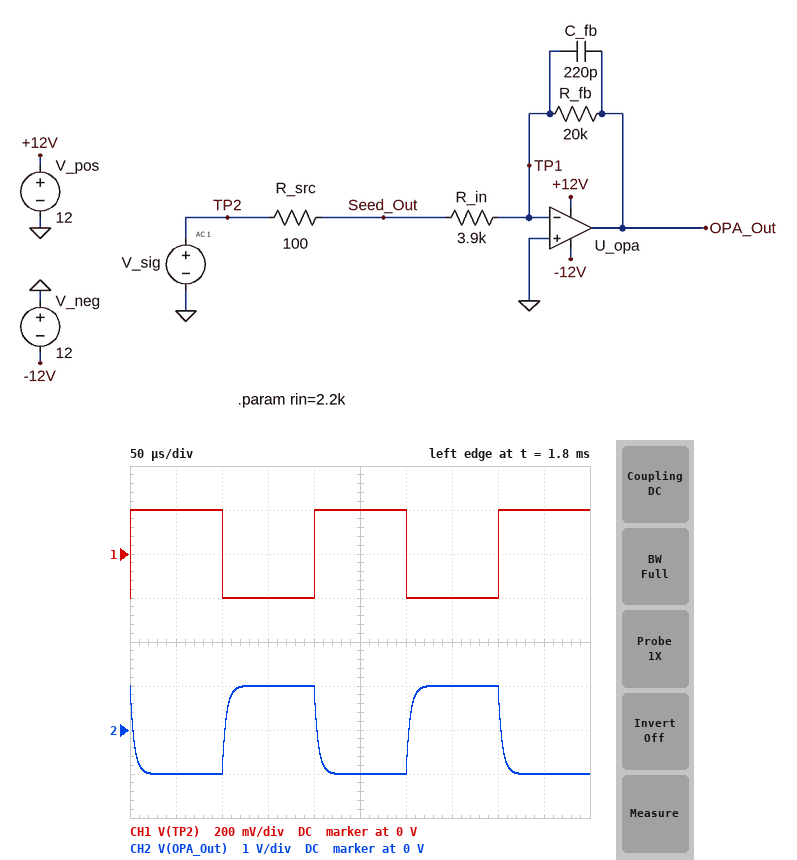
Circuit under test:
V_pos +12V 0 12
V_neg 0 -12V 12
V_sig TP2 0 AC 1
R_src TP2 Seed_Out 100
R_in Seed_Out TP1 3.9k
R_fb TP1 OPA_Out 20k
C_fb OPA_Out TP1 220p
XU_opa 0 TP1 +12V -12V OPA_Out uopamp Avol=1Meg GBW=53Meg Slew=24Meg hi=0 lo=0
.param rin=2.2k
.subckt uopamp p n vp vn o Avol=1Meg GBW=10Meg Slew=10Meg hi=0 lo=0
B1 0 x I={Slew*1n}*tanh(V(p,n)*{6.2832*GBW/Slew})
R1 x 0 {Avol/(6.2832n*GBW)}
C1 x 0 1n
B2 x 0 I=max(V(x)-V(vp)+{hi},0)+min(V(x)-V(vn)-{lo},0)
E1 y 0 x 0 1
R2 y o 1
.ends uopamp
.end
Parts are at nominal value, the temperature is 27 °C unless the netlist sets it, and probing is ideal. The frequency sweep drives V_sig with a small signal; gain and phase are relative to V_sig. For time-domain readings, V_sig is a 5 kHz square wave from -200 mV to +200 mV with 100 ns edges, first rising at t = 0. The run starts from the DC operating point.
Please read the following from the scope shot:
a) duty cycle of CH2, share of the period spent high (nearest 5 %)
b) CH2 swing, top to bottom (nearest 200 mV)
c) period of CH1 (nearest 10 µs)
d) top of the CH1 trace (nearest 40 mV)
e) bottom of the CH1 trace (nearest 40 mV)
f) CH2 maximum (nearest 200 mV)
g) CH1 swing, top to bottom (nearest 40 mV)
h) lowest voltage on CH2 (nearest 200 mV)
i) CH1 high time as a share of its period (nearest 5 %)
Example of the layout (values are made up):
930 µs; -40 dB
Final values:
50 %; 2.0 V; 200 µs; 200 mV; -200 mV; 1.0 V; 400 mV; -1.0 V; 50 %
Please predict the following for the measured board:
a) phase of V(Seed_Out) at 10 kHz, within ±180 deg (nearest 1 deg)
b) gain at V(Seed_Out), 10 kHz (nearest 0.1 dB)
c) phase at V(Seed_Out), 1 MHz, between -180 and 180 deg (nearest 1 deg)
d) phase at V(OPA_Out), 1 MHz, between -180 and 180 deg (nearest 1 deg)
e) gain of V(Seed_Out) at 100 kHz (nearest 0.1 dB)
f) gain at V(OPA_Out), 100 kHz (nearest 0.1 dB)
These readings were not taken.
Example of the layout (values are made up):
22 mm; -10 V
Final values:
0 deg; -0.2 dB; 0 deg; 91 deg; -0.2 dB; 4.6 dB
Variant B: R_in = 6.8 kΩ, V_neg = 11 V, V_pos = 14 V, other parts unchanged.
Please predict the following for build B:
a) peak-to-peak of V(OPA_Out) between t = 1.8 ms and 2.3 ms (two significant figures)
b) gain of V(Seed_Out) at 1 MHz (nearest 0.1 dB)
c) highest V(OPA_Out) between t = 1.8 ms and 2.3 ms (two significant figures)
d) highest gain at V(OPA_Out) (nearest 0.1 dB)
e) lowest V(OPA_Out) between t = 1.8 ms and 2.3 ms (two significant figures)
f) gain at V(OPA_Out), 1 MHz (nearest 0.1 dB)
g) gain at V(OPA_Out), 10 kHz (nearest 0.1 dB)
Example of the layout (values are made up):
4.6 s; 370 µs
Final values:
1.2 V; -0.1 dB; 580 mV; 9.2 dB; -580 mV; -19.6 dB; 8.9 dB
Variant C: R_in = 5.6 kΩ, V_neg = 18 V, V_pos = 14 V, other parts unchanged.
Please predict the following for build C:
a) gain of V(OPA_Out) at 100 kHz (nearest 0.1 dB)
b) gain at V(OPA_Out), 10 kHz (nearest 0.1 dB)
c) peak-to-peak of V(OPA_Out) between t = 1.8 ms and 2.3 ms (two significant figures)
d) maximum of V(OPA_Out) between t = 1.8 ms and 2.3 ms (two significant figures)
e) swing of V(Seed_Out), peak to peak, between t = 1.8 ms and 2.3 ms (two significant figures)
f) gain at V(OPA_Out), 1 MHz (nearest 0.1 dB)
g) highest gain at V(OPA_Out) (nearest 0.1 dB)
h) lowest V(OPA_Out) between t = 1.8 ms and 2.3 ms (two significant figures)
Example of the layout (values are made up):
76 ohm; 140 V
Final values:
1.5 dB; 10.6 dB; 1.4 V; 700 mV; 390 mV; -18.0 dB; 10.9 dB; -700 mV
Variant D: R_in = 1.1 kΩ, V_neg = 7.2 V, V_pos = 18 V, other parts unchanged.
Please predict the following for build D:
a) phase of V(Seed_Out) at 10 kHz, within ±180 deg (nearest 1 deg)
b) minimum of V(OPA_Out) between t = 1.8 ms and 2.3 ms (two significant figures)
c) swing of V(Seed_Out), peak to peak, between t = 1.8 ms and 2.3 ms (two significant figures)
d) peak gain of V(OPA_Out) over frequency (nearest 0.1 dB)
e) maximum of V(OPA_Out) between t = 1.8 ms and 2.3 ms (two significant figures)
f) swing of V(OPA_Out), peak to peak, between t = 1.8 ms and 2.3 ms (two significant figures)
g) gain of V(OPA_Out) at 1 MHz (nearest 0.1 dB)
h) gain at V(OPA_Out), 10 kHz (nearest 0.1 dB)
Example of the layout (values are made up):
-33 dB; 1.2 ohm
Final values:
0 deg; -3.3 V; 370 mV; 24.4 dB; 3.3 V; 6.7 V; -4.5 dB; 24.1 dB
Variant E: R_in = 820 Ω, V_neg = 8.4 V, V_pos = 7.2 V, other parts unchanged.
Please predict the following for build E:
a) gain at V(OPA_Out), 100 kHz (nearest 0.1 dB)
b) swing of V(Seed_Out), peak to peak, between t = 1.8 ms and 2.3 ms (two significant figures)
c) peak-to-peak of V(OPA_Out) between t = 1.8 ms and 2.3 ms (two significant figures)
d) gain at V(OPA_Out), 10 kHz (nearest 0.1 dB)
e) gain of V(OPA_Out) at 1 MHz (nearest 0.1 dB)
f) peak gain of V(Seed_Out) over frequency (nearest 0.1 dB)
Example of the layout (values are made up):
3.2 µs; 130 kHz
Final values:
17.3 dB; 360 mV; 8.7 V; 26.4 dB; -2.2 dB; -1.0 dB
